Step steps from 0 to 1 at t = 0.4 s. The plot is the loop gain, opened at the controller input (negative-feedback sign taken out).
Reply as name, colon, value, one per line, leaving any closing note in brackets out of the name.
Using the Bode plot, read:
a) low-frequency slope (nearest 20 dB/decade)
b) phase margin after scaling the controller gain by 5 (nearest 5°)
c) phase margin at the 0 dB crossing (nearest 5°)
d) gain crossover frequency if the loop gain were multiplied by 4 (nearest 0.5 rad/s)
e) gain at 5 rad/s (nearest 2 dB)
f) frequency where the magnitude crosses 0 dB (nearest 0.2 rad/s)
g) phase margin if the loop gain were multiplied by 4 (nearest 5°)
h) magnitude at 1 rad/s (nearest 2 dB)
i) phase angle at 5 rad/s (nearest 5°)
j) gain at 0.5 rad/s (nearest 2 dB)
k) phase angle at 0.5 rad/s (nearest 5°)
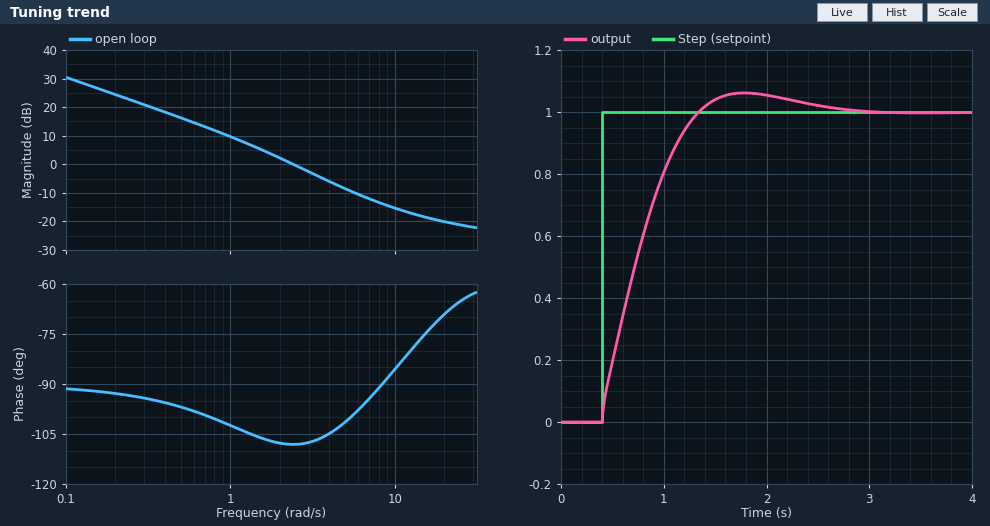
low-frequency slope: -20 dB/decade
phase margin after scaling the controller gain by 5: 90°
phase margin at the 0 dB crossing: 70°
gain crossover frequency if the loop gain were multiplied by 4: 7.0 rad/s
gain at 5 rad/s: -8 dB
frequency where the magnitude crosses 0 dB: 2.4 rad/s
phase margin if the loop gain were multiplied by 4: 85°
magnitude at 1 rad/s: 10 dB
phase angle at 5 rad/s: -100°
gain at 0.5 rad/s: 16 dB
phase angle at 0.5 rad/s: -95°
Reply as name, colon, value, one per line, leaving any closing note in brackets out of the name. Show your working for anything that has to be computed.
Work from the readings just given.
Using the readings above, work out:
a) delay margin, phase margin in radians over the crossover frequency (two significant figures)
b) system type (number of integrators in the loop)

delay margin, phase margin in radians over the crossover frequency: 70 × π / 180 / 2.4 = 0.51 s
system type: 1
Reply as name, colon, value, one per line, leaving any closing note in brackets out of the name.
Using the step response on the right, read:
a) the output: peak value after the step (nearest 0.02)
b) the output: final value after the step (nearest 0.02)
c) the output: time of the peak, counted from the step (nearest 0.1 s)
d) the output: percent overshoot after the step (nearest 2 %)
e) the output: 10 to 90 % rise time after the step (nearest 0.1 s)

the output: peak value after the step: 1.06
the output: final value after the step: 1.00
the output: time of the peak, counted from the step: 1.4 s
the output: percent overshoot after the step: 6 %
the output: 10 to 90 % rise time after the step: 0.7 s
